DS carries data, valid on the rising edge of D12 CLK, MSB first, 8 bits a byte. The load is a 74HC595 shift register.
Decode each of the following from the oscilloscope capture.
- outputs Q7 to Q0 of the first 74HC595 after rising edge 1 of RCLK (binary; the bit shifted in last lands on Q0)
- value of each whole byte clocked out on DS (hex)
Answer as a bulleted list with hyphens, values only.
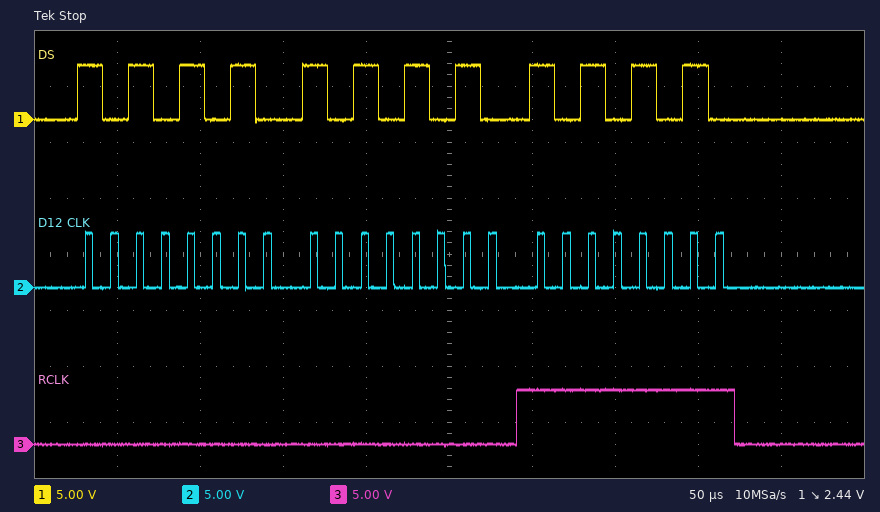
- 10101010
- 0xAA 0xAA 0xAA
